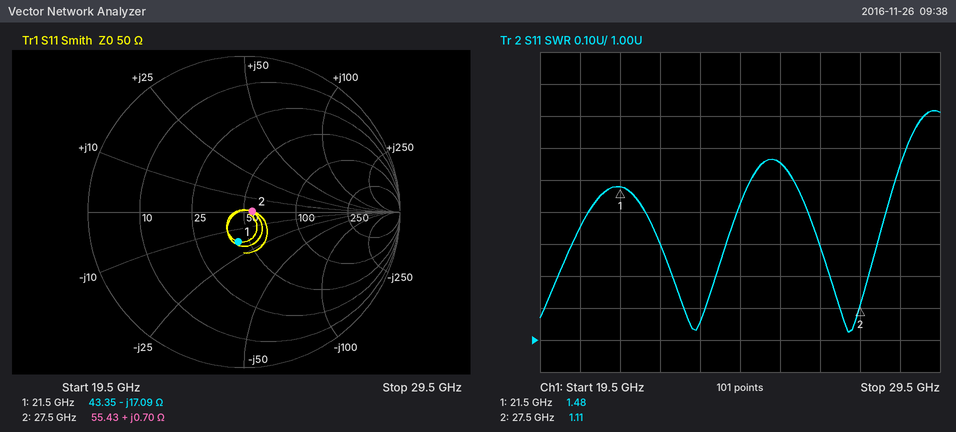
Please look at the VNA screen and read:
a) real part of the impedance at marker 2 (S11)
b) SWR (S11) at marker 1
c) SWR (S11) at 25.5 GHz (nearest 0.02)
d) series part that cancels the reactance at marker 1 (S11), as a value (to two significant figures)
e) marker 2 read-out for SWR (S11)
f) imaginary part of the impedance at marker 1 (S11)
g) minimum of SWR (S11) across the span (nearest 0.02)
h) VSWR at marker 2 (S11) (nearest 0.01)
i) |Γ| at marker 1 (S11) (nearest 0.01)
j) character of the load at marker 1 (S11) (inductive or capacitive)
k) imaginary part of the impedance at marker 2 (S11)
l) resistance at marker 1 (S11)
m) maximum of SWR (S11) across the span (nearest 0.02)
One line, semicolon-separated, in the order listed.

55.43 Ω; 1.48; 1.56; 130 pH; 1.11; -17.09 Ω; 1.02; 1.11; 0.19; capacitive; +0.70 Ω; 43.35 Ω; 1.72
